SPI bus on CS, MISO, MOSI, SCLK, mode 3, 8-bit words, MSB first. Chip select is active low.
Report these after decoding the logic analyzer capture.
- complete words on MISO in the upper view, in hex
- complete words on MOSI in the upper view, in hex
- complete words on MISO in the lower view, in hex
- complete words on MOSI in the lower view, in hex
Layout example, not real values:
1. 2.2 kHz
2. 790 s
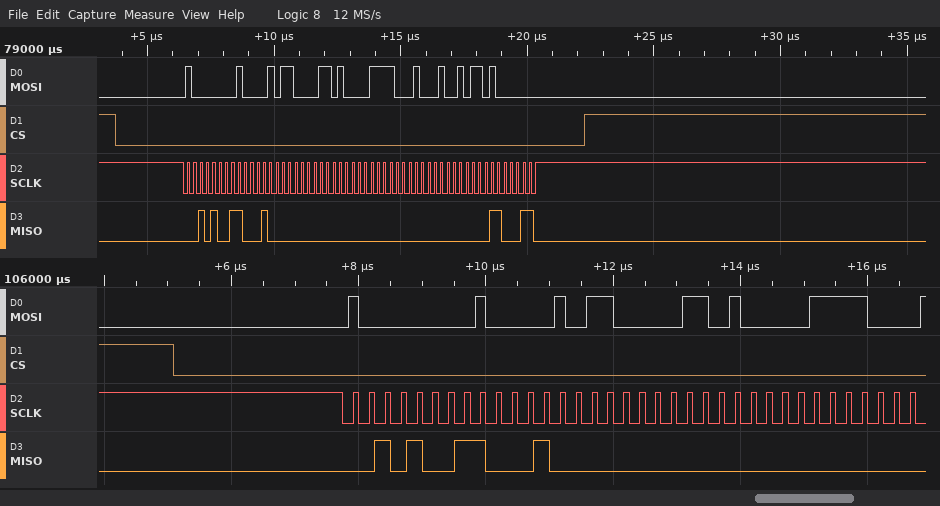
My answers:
1. 29, 88, 00, 00, 00, 00, C6
2. 80, 85, 86, 87, 88, 96, 80
3. 29, 88, 00, 00
4. 80, 85, 86, 87
